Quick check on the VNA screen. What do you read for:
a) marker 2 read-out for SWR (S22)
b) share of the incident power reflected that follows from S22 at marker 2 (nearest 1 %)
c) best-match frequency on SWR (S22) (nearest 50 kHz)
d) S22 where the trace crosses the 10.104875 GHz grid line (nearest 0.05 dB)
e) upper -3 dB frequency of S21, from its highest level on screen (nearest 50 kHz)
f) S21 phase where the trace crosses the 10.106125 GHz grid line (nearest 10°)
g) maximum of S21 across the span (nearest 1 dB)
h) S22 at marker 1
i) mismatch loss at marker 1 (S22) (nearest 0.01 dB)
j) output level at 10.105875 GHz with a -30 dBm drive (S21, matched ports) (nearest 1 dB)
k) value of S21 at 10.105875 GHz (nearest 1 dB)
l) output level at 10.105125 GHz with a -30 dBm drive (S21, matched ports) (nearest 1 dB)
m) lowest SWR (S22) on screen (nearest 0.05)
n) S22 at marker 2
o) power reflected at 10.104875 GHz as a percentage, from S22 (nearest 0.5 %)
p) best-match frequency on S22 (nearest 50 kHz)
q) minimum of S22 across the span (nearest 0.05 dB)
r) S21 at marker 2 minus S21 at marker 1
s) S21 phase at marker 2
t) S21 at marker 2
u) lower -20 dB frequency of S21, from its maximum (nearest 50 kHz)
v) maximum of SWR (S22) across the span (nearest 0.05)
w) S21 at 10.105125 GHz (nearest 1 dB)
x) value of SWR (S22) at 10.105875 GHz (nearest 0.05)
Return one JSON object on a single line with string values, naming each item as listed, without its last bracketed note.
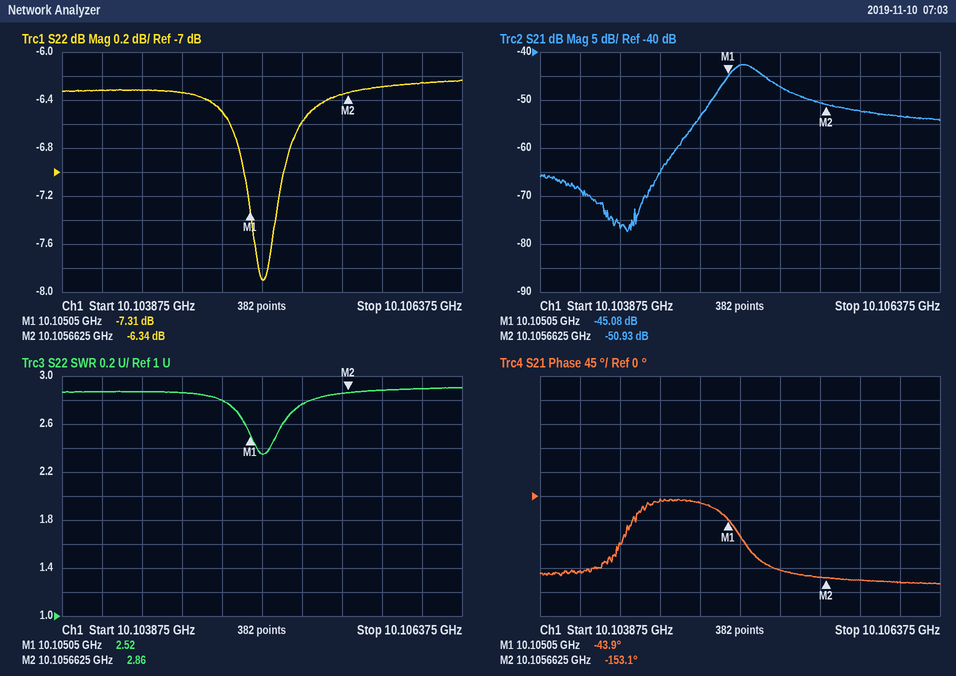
{"marker 2 read-out for SWR": "2.86", "share of the incident power reflected that follows from S22 at marker 2": "23 %", "best-match frequency on SWR (S22)": "10.10515 GHz", "S22 where the trace crosses the 10.104875 GHz grid line": "-6.50 dB", "upper -3 dB frequency of S21, from its highest level on screen": "10.10530 GHz", "S21 phase where the trace crosses the 10.106125 GHz grid line": "-160°", "maximum of S21 across the span": "-43 dB", "S22 at marker 1": "-7.31 dB", "mismatch loss at marker 1 (S22)": "0.89 dB", "output level at 10.105875 GHz with a -30 dBm drive (S21, matched ports)": "-82 dBm", "value of S21 at 10.105875 GHz": "-52 dB", "output level at 10.105125 GHz with a -30 dBm drive (S21, matched ports)": "-73 dBm", "lowest SWR (S22) on screen": "2.35", "S22 at marker 2": "-6.34 dB", "power reflected at 10.104875 GHz as a percentage, from S22": "22.5 %", "best-match frequency on S22": "10.10515 GHz", "minimum of S22 across the span": "-7.90 dB", "S21 at marker 2 minus S21 at marker 1": "-5.85 dB", "S21 phase at marker 2": "-153.1°", "S21 at marker 2": "-50.93 dB", "lower -20 dB frequency of S21, from its maximum": "10.10465 GHz", "maximum of SWR (S22) across the span": "2.90", "S21 at 10.105125 GHz": "-43 dB", "value of SWR (S22) at 10.105875 GHz": "2.90"}
